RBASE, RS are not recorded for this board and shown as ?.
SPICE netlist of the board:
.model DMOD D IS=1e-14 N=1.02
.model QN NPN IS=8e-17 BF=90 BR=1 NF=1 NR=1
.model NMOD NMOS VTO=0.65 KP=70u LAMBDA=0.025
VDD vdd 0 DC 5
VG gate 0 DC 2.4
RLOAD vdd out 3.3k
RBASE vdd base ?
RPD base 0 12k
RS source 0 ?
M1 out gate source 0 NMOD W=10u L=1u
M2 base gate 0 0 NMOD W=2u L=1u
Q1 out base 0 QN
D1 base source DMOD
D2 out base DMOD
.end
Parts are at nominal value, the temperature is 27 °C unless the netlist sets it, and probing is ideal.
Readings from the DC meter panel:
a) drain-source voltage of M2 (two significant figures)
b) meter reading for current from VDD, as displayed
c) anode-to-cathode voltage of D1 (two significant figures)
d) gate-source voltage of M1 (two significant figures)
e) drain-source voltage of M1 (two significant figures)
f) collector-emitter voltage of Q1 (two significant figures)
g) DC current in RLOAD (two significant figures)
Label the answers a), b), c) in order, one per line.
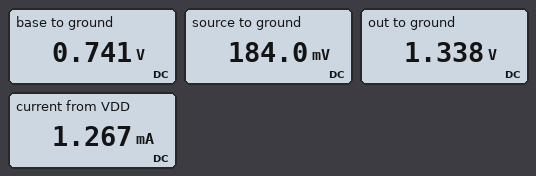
a) 740 mV
b) 1.267 mA
c) 560 mV
d) 2.2 V
e) 1.2 V
f) 1.3 V
g) 1.1 mA
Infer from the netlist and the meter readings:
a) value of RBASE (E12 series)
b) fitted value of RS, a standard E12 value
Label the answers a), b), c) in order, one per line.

a) 27 kΩ
b) 220 Ω
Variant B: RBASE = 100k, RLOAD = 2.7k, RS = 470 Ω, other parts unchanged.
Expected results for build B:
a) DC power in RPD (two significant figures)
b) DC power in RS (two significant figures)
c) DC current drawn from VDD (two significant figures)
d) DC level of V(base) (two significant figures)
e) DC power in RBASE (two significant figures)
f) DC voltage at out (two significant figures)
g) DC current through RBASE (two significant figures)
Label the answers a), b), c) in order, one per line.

a) 48 µW
b) 220 µW
c) 1.4 mA
d) 760 mV
e) 180 µW
f) 1.4 V
g) 42 µA
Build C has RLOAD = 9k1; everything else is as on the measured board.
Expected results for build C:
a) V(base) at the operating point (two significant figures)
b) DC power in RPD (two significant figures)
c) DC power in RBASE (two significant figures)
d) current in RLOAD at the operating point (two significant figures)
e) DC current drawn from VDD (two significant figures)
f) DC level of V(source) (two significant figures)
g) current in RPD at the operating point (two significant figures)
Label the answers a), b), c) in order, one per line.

a) 560 mV
b) 26 µW
c) 730 µW
d) 480 µA
e) 650 µA
f) 110 mV
g) 47 µA
